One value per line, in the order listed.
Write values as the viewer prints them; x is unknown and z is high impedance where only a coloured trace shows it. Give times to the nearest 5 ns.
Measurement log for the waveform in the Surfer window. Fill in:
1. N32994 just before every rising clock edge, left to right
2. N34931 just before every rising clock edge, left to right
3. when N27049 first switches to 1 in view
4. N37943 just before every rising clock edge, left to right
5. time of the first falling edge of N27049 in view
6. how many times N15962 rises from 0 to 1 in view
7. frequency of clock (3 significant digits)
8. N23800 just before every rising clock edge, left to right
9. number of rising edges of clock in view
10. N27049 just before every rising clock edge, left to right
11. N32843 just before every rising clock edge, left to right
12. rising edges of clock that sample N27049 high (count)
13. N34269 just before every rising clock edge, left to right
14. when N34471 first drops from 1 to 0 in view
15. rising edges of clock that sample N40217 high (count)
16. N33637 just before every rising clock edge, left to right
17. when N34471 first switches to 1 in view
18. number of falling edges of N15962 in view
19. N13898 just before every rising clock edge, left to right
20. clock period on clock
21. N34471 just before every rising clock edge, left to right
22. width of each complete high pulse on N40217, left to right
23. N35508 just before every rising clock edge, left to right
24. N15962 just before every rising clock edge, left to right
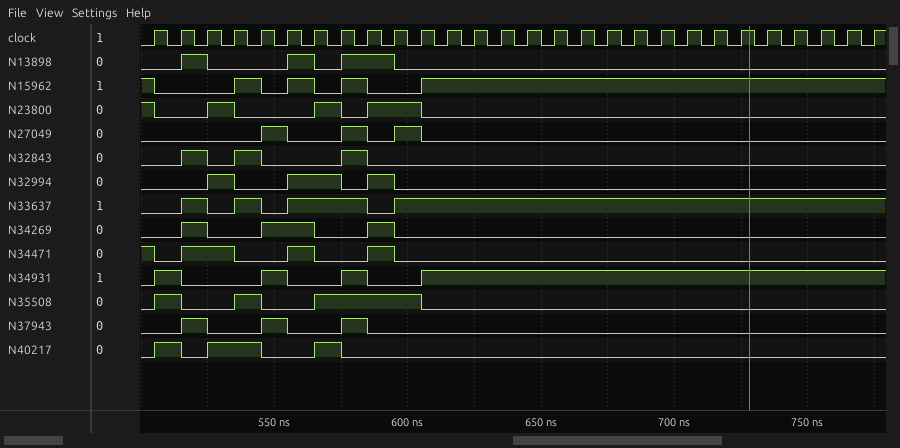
0 0 0 1 0 0 1 1 0 1 0 0 0 0 0 0 0 0 0 0 0 0 0 0 0 0 0 0
0 1 0 0 0 1 0 0 1 0 0 1 1 1 1 1 1 1 1 1 1 1 1 1 1 1 1 1
545 ns
0 0 1 0 0 1 0 0 1 0 0 0 0 0 0 0 0 0 0 0 0 0 0 0 0 0 0 0
555 ns
4
100 MHz
1 0 0 1 0 0 0 1 0 1 1 0 0 0 0 0 0 0 0 0 0 0 0 0 0 0 0 0
28
0 0 0 0 0 1 0 0 1 0 1 0 0 0 0 0 0 0 0 0 0 0 0 0 0 0 0 0
0 0 1 0 1 0 0 0 1 0 0 0 0 0 0 0 0 0 0 0 0 0 0 0 0 0 0 0
3
0 0 1 0 0 1 1 0 0 1 0 0 0 0 0 0 0 0 0 0 0 0 0 0 0 0 0 0
505 ns
4
0 0 1 0 1 0 1 1 1 0 1 1 1 1 1 1 1 1 1 1 1 1 1 1 1 1 1 1
515 ns
4
0 0 1 0 0 0 1 0 1 1 0 0 0 0 0 0 0 0 0 0 0 0 0 0 0 0 0 0
10 ns
1 0 1 1 0 0 1 0 0 1 0 0 0 0 0 0 0 0 0 0 0 0 0 0 0 0 0 0
10 ns, 20 ns, 10 ns
0 1 0 0 1 0 0 1 1 1 1 0 0 0 0 0 0 0 0 0 0 0 0 0 0 0 0 0
1 0 0 0 1 0 1 0 1 0 0 1 1 1 1 1 1 1 1 1 1 1 1 1 1 1 1 1
